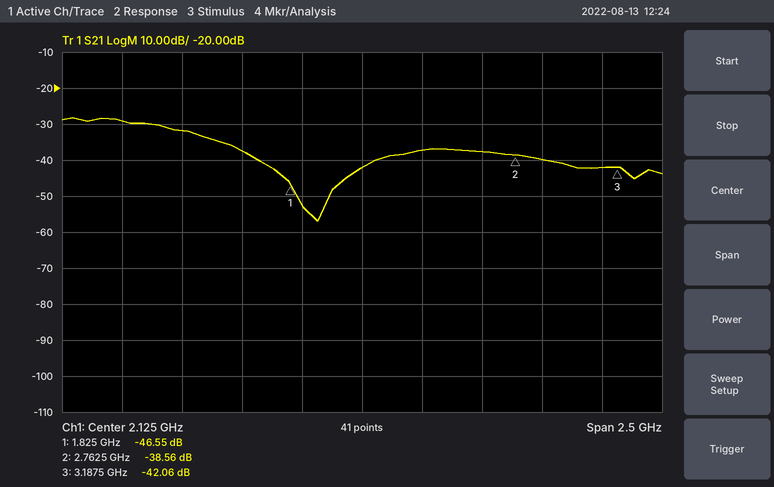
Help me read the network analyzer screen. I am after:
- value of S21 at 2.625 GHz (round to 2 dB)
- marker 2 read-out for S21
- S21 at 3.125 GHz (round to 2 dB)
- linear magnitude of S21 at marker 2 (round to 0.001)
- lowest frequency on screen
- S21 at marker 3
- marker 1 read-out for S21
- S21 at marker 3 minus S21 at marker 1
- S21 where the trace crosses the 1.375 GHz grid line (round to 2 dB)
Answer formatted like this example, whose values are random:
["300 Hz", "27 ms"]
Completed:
["-38 dB", "-38.56 dB", "-42 dB", "0.012", "875 MHz", "-42.06 dB", "-46.55 dB", "4.49 dB", "-32 dB"]
